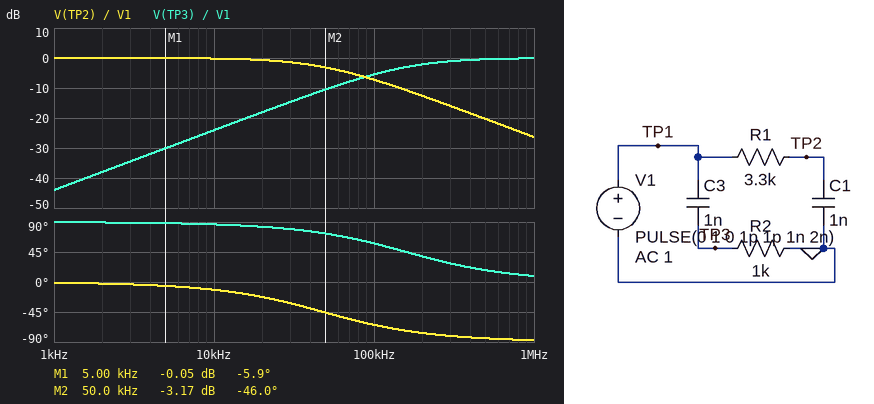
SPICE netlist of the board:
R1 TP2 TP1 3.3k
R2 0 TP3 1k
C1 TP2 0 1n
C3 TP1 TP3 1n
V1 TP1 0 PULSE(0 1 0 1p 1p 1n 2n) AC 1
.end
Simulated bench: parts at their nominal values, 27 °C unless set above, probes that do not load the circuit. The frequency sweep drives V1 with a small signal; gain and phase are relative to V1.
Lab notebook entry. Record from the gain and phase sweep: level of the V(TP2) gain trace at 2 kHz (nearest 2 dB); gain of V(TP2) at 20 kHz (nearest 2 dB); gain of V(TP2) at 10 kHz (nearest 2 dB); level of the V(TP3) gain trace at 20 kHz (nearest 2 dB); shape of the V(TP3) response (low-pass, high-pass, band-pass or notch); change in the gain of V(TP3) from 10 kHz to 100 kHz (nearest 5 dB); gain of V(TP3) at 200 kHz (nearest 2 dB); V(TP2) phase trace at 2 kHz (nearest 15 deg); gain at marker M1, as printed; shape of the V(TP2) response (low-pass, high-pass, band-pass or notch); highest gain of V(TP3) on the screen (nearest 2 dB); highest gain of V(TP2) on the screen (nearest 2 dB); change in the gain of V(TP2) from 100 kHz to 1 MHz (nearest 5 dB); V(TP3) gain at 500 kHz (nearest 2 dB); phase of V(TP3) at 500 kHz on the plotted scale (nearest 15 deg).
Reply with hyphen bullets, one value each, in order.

- 0 dB
- 0 dB
- 0 dB
- -18 dB
- high-pass
- 20 dB
- -2 dB
- 0 deg
- -0.05 dB
- low-pass
- 0 dB
- 0 dB
- -20 dB
- 0 dB
- 15 deg
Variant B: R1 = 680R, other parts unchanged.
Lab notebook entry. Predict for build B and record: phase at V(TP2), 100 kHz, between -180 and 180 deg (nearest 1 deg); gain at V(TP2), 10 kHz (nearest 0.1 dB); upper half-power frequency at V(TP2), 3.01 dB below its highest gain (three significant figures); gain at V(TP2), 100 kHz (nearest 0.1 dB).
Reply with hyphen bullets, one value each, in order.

- -23 deg
- 0 dB
- 234 kHz
- -0.7 dB
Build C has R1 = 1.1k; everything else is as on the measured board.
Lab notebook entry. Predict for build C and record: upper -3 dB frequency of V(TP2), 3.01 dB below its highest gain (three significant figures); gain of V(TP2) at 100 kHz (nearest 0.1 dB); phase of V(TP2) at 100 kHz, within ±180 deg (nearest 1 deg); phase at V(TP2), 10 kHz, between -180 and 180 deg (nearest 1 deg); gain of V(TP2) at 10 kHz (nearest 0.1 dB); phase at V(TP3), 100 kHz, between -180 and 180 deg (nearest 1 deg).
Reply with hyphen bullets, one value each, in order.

- 145 kHz
- -1.7 dB
- -35 deg
- -4 deg
- 0 dB
- 58 deg
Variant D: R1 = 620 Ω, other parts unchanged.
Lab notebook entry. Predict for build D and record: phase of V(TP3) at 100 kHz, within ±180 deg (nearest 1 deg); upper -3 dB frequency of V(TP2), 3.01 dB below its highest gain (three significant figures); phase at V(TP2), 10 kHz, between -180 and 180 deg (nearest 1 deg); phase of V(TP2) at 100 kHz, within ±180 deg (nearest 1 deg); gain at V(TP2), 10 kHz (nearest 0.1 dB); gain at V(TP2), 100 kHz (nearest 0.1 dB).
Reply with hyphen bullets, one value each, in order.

- 58 deg
- 257 kHz
- -2 deg
- -21 deg
- 0 dB
- -0.6 dB
